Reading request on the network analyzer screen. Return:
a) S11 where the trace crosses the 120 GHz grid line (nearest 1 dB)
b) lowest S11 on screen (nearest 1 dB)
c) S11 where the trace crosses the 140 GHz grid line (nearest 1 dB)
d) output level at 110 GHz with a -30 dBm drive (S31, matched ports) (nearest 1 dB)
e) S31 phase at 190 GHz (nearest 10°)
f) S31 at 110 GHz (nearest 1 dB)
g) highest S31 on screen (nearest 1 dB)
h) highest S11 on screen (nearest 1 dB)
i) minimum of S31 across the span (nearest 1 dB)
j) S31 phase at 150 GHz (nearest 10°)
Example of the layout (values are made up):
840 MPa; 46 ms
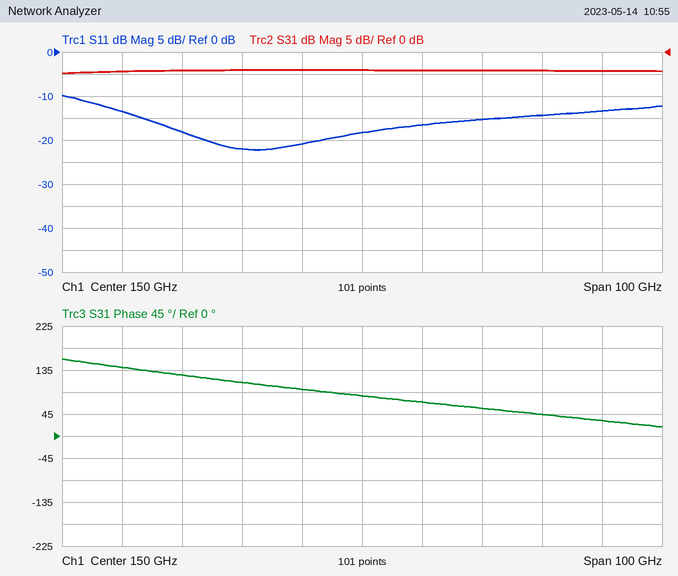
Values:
-18 dB; -22 dB; -21 dB; -34 dBm; 30°; -4 dB; -4 dB; -10 dB; -5 dB; 80°
